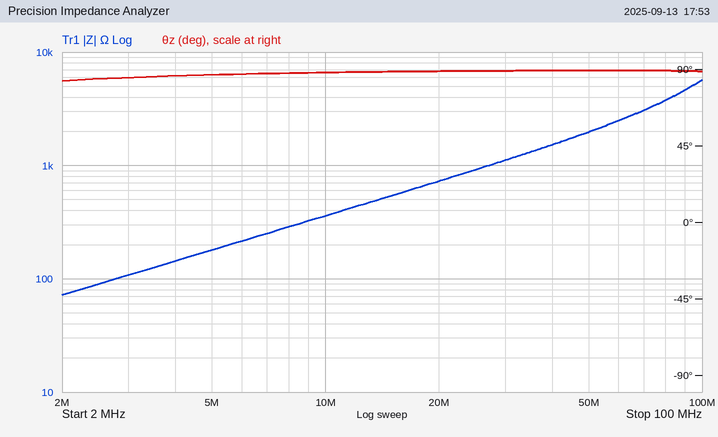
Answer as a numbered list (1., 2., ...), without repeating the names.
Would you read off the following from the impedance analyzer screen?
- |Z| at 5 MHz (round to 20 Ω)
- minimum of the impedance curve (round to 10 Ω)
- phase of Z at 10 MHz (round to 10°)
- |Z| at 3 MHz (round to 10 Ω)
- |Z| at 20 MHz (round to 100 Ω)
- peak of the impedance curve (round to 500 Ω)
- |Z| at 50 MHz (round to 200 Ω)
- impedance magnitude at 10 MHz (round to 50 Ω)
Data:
1. 180 Ω
2. 70 Ω
3. 90°
4. 110 Ω
5. 700 Ω
6. 5.5 kΩ
7. 2.0 kΩ
8. 350 Ω
